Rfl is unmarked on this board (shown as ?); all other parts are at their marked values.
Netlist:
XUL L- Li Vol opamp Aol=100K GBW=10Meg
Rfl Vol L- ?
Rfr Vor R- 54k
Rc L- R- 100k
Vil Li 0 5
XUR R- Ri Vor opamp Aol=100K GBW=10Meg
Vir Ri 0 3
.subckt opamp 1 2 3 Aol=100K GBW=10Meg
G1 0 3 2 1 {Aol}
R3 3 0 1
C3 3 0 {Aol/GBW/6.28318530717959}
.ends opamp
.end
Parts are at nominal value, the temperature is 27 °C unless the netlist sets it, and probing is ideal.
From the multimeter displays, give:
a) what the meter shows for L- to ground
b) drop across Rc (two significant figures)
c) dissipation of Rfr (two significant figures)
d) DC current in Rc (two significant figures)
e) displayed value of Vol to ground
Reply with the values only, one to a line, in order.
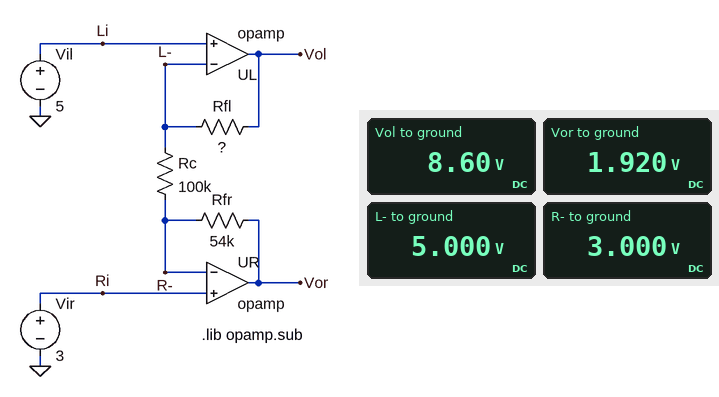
5.000 V
2.0 V
22 µW
20 µA
8.60 V
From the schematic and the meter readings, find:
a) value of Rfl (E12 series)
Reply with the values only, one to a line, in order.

180 kΩ
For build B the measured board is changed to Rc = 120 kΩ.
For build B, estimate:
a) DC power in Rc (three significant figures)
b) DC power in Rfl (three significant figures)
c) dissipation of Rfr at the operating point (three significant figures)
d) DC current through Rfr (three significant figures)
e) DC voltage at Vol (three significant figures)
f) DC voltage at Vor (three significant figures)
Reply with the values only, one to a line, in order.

33.3 µW
50.0 µW
15.0 µW
16.7 µA
8.00 V
2.10 V
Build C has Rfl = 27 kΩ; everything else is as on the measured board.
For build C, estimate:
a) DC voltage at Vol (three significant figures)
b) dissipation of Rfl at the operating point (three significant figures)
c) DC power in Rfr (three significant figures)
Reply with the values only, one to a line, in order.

5.54 V
10.8 µW
21.6 µW
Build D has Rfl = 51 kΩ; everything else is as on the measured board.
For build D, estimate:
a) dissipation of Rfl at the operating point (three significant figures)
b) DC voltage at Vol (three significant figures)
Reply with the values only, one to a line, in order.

20.4 µW
6.02 V
